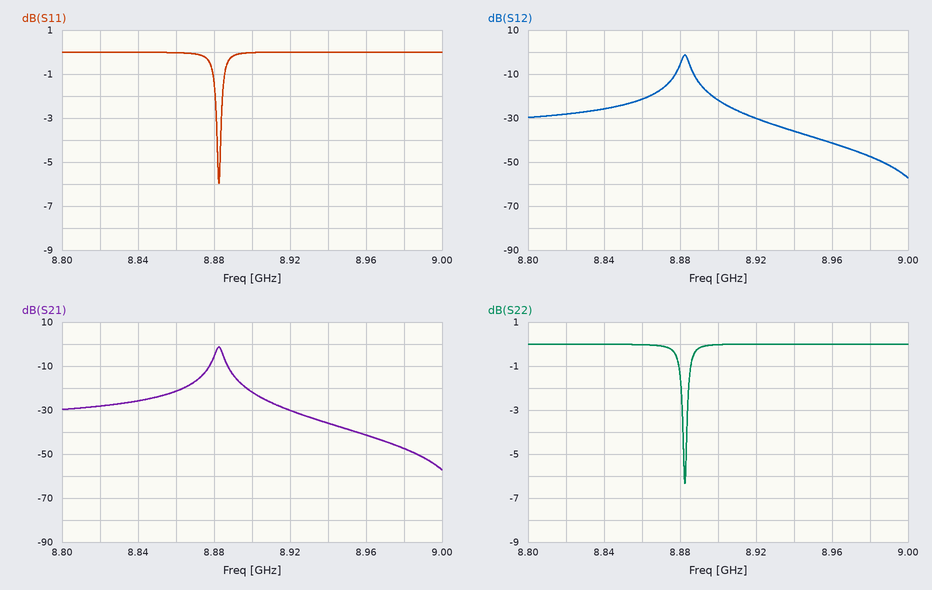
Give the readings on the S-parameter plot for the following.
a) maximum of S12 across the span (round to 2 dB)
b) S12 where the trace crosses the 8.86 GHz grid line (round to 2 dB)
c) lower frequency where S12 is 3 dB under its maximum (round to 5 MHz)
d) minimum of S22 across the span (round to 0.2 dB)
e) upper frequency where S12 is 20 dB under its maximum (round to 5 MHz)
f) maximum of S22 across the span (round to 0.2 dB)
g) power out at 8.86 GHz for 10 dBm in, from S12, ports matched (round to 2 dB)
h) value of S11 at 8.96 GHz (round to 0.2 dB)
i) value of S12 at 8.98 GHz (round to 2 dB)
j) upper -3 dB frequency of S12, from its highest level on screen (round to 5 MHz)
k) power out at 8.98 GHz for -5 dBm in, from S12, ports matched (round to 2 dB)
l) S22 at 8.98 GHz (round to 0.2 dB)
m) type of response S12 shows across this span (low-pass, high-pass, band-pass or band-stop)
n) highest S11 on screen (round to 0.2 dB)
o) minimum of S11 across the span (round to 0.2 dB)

-2 dB
-22 dB
8.880 GHz
-6.4 dB
8.900 GHz
0.0 dB
-12 dBm
0.0 dB
-48 dB
8.885 GHz
-52 dBm
0.0 dB
band-pass
0.0 dB
-6.0 dB
